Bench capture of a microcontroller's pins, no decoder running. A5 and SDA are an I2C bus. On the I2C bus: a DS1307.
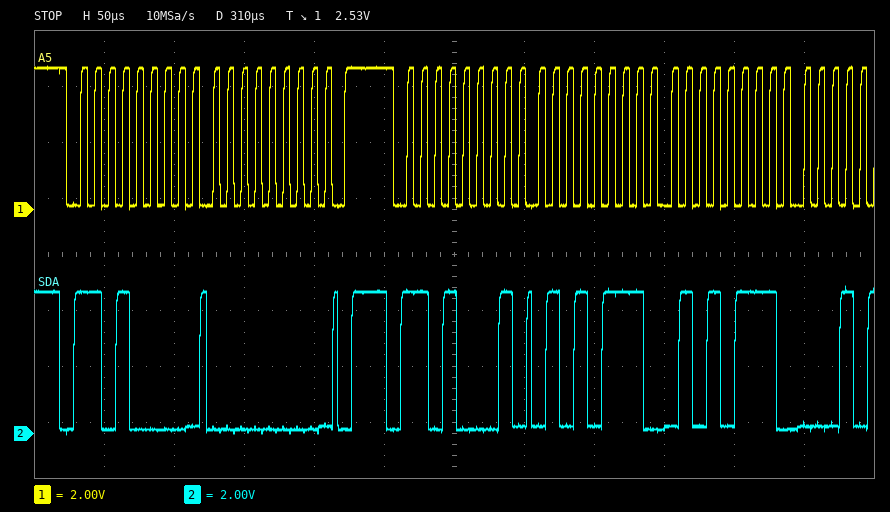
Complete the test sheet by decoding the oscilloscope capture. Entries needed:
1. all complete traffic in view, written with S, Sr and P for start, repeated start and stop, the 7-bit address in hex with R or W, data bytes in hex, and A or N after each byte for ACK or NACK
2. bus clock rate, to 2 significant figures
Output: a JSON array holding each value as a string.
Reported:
["S 68W A 00 A P S 68R A 57 A 57 A", "100 kHz"]
